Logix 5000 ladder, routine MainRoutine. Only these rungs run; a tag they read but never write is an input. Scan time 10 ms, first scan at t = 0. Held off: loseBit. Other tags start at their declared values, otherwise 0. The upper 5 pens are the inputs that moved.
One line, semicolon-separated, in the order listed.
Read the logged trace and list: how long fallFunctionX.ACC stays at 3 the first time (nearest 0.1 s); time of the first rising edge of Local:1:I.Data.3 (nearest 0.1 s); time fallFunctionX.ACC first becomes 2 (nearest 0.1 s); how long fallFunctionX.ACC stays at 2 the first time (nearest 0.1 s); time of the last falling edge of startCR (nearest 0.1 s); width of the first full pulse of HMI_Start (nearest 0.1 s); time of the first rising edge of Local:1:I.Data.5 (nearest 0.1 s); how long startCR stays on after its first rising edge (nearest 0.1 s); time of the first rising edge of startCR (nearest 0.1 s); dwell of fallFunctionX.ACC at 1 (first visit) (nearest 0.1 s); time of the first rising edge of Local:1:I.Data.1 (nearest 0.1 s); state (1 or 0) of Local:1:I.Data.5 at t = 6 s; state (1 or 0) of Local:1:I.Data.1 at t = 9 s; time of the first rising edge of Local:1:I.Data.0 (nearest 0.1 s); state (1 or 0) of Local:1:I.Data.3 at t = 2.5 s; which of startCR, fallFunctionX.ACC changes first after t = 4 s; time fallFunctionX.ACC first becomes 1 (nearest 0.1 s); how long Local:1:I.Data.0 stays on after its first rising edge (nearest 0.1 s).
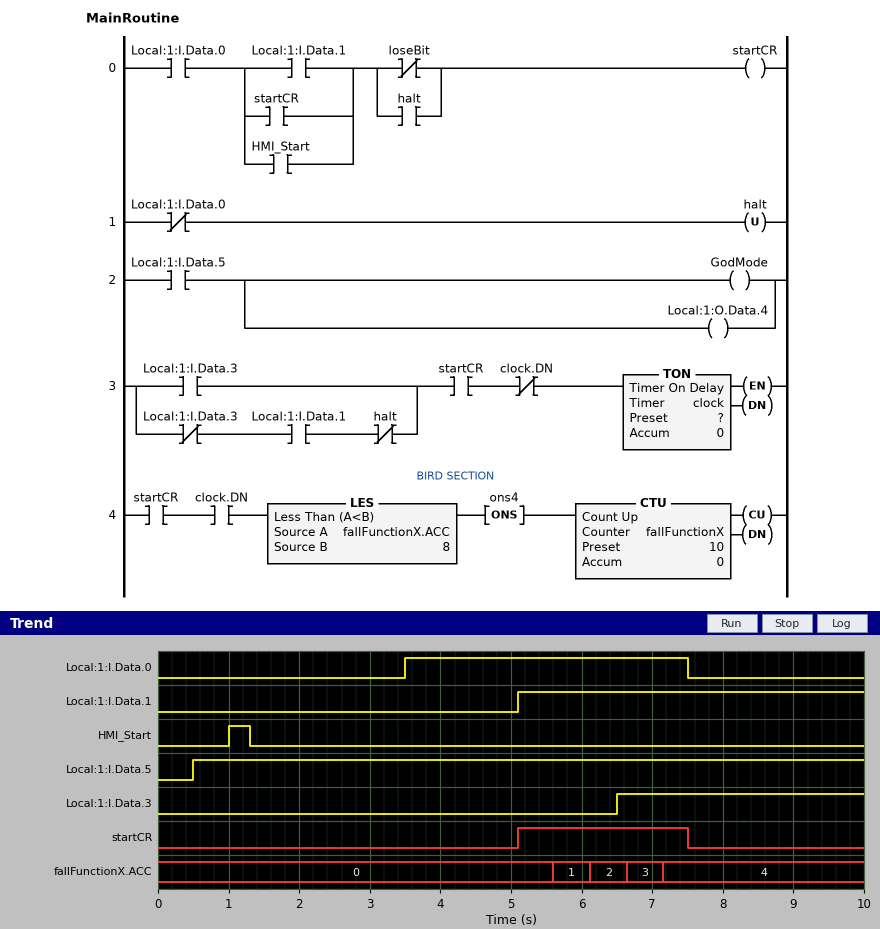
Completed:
0.5 s; 6.5 s; 6.1 s; 0.5 s; 7.5 s; 0.3 s; 0.5 s; 2.4 s; 5.1 s; 0.5 s; 5.1 s; 1; 1; 3.5 s; 0; startCR; 5.6 s; 4.0 s
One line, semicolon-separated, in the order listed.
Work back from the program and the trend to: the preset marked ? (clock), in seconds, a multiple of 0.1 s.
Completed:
0.5 s
